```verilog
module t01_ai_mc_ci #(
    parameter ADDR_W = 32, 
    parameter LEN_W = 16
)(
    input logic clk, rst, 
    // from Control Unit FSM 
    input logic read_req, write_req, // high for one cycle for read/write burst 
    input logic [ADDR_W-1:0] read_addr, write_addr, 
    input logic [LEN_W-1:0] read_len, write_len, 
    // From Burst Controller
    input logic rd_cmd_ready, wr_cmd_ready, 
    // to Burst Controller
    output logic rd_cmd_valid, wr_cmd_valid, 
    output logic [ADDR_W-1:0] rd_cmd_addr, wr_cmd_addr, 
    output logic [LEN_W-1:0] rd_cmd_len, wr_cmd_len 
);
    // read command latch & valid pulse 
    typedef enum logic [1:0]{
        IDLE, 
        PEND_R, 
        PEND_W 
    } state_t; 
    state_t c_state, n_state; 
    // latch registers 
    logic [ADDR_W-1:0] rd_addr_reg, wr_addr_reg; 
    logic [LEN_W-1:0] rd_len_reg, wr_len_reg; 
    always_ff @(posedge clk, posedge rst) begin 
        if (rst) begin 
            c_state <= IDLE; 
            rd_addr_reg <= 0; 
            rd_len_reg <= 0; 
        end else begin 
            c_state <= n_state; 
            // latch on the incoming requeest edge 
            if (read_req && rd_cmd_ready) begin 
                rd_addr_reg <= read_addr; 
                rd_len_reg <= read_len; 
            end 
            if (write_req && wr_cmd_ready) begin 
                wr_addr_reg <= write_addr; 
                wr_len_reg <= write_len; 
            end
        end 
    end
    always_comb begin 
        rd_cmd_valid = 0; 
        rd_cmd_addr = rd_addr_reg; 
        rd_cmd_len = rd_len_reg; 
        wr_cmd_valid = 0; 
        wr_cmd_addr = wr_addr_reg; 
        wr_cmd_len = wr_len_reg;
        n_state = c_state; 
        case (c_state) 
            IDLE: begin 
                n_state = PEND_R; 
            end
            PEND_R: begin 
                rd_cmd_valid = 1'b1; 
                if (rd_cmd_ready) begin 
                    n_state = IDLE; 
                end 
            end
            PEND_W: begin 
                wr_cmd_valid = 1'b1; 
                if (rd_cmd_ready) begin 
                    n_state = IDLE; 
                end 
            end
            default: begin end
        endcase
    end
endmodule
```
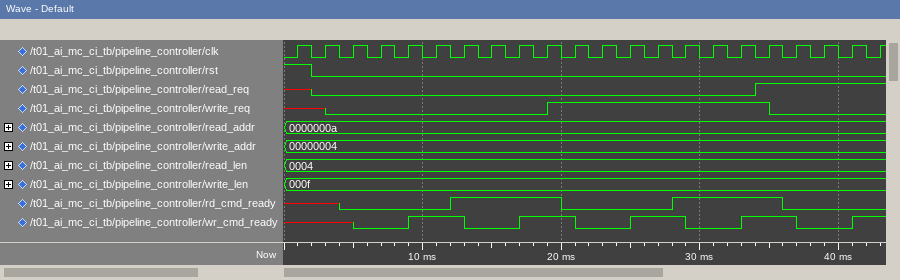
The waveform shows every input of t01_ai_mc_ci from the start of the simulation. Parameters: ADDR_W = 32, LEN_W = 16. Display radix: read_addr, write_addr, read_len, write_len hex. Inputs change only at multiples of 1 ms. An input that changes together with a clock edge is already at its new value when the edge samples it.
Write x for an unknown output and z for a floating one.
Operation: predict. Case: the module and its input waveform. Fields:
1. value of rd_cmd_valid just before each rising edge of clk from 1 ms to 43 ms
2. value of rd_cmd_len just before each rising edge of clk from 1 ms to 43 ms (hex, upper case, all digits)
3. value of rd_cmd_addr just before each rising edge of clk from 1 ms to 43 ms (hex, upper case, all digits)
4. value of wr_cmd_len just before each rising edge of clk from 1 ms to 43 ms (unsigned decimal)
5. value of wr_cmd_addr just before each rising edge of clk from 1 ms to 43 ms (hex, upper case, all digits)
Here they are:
0 0 1 1 1 1 1 0 1 0 1 1 1 1 1 0 1 0 1 1 1 1
0000, 0000, 0000, 0000, 0000, 0000, 0000, 0000, 0000, 0000, 0000, 0000, 0000, 0000, 0000, 0000, 0000, 0000, 0004, 0004, 0004, 0004
00000000, 00000000, 00000000, 00000000, 00000000, 00000000, 00000000, 00000000, 00000000, 00000000, 00000000, 00000000, 00000000, 00000000, 00000000, 00000000, 00000000, 00000000, 0000000A, 0000000A, 0000000A, 0000000A
x, x, x, x, x, x, x, x, x, x, 15, 15, 15, 15, 15, 15, 15, 15, 15, 15, 15, 15
x, x, x, x, x, x, x, x, x, x, 00000004, 00000004, 00000004, 00000004, 00000004, 00000004, 00000004, 00000004, 00000004, 00000004, 00000004, 00000004
